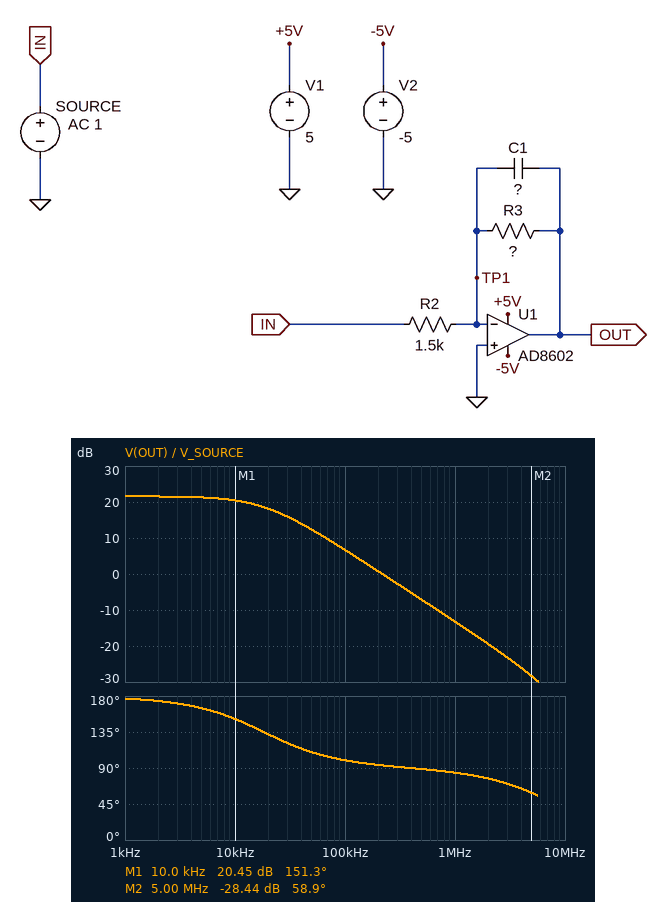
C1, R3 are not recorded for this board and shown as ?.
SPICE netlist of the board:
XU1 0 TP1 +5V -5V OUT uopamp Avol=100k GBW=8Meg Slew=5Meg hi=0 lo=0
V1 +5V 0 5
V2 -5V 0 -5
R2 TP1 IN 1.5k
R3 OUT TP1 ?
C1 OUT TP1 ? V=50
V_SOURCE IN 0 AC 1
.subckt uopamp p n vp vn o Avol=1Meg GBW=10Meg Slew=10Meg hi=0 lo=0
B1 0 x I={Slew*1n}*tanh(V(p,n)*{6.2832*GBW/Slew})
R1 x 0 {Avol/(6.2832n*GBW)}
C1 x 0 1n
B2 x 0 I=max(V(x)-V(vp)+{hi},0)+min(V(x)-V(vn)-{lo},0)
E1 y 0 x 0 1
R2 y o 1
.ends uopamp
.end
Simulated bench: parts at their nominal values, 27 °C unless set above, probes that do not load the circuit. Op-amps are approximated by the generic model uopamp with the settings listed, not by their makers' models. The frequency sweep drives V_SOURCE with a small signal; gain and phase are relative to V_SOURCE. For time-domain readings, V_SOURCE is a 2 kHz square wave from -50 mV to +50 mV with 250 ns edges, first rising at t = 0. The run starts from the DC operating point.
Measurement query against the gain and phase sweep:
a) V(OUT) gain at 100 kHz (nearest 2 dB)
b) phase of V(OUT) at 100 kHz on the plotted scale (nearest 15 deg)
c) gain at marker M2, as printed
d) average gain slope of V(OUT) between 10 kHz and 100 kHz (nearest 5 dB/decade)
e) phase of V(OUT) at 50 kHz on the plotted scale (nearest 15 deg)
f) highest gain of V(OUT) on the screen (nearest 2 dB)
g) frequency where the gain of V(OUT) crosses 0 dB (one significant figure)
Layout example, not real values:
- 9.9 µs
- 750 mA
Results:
- 6 dB
- 105 deg
- -28.44 dB
- -15 dB/decade
- 105 deg
- 22 dB
- 200 kHz
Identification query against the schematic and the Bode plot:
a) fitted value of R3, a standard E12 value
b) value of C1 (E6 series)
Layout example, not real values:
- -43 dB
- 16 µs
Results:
- 18 kΩ
- 470 pF
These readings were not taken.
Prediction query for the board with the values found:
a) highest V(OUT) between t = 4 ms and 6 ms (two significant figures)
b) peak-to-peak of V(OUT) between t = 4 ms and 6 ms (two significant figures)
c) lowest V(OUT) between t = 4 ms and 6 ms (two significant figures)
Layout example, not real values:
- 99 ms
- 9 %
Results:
- 600 mV
- 1.2 V
- -600 mV
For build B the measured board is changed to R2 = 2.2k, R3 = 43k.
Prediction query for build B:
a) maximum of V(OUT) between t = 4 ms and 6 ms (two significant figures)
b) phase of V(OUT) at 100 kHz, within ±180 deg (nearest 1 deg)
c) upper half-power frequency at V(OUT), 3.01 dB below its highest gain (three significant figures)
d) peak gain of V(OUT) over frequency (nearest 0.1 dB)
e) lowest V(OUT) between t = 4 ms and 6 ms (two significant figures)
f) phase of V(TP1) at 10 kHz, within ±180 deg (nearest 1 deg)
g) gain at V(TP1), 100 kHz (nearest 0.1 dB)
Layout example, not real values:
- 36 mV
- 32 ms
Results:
- 980 mV
- 94 deg
- 7.73 kHz
- 25.8 dB
- -980 mV
- 37 deg
- -34.5 dB
